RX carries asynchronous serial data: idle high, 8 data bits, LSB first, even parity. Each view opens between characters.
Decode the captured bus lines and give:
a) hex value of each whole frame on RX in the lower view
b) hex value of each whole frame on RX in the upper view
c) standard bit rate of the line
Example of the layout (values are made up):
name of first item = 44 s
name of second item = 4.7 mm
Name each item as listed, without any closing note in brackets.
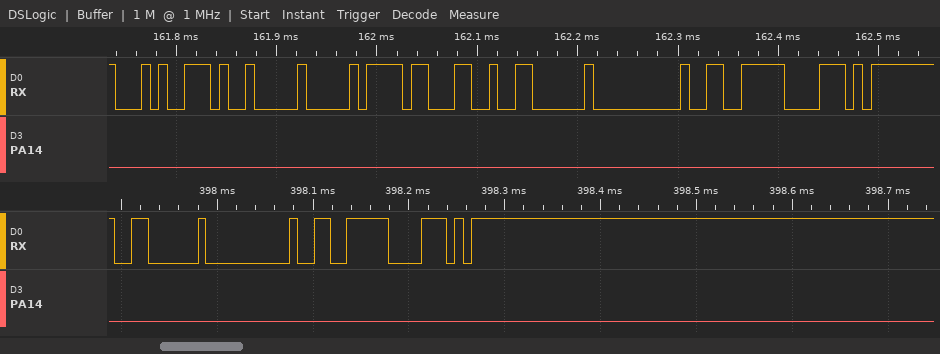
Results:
hex value of each whole frame on RX in the lower view = 06, 00, E6, B8
hex value of each whole frame on RX in the upper view = 94, 09, D0, 63, 06, 00, E6, B8
standard bit rate of the line = 115200 baud
